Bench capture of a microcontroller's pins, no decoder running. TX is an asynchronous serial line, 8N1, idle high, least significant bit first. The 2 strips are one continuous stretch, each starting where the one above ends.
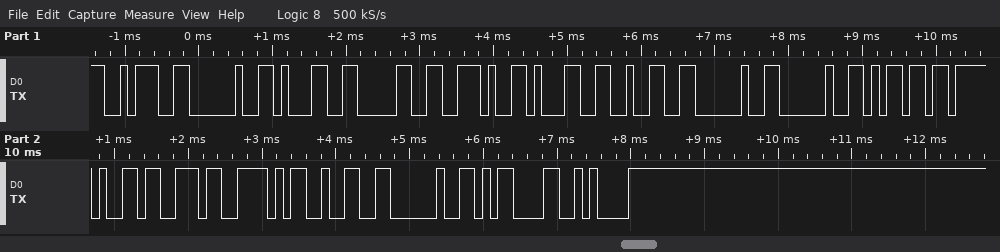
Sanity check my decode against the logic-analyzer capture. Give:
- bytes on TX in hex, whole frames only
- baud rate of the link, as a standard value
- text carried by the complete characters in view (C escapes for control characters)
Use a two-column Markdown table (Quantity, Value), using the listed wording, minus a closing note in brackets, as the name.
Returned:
| Quantity | Value |
|---|---|
| bytes on TX in hex, whole frames only | 0x3A 0x20 0x31 0x30 0x2E 0x31 0x32 0x20 0x20 0x6D 0x2F 0x73 0x5E 0x32 0x20 0x0D 0x0A |
| baud rate of the link, as a standard value | 9600 baud |
| text carried by the complete characters in view | ": 10.12  m/s^2 \r\n" |
